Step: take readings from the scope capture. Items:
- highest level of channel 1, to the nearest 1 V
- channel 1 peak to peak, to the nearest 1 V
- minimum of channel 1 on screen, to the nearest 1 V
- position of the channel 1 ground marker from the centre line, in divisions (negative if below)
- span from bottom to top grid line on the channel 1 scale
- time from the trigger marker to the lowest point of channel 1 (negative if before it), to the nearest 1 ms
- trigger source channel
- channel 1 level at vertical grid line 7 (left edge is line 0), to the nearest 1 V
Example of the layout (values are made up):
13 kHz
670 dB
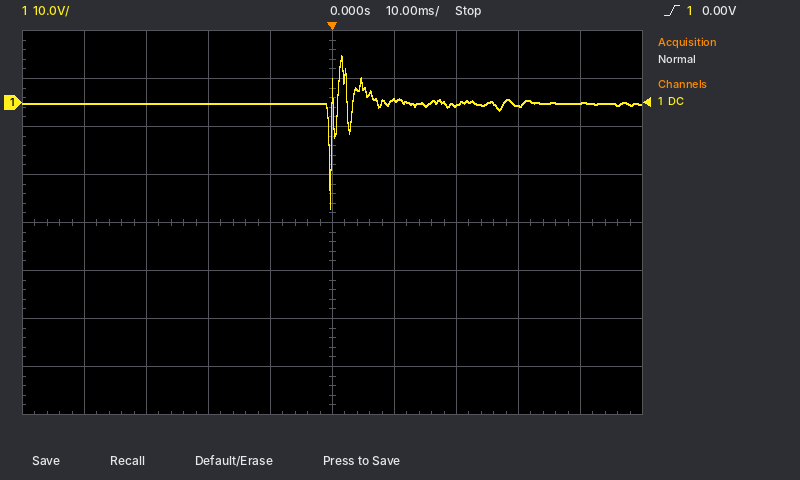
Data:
10 V
32 V
-22 V
+2.5 div
80 V
0 ms
channel 1
-1 V
